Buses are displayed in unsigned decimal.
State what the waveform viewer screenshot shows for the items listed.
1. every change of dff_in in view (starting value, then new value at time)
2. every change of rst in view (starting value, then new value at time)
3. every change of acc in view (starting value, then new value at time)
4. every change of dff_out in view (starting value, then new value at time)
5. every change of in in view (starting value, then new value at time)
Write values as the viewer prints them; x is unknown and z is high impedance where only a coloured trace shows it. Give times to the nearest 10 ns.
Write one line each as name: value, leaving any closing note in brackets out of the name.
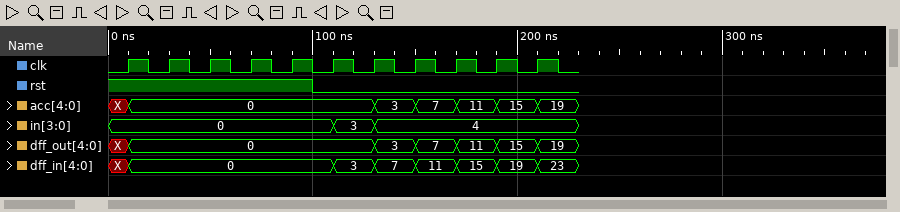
every change of dff_in in view: X, 0 at 10 ns, 3 at 110 ns, 7 at 130 ns, 11 at 150 ns, 15 at 170 ns, 19 at 190 ns, 23 at 210 ns
every change of rst in view: 1, 0 at 100 ns
every change of acc in view: X, 0 at 10 ns, 3 at 130 ns, 7 at 150 ns, 11 at 170 ns, 15 at 190 ns, 19 at 210 ns
every change of dff_out in view: X, 0 at 10 ns, 3 at 130 ns, 7 at 150 ns, 11 at 170 ns, 15 at 190 ns, 19 at 210 ns
every change of in in view: 0, 3 at 110 ns, 4 at 130 ns
